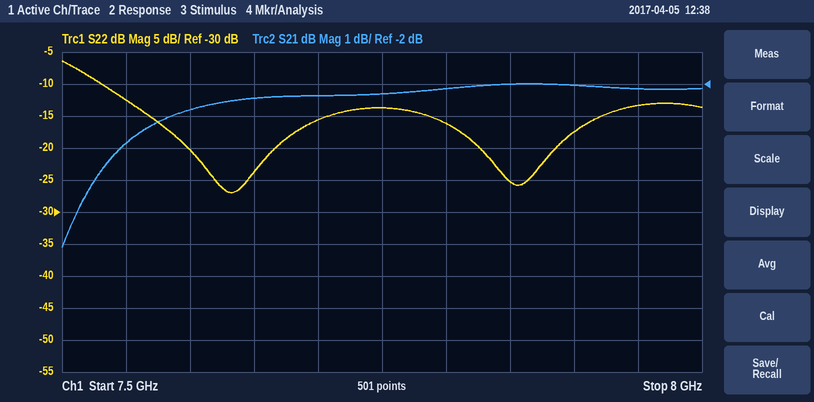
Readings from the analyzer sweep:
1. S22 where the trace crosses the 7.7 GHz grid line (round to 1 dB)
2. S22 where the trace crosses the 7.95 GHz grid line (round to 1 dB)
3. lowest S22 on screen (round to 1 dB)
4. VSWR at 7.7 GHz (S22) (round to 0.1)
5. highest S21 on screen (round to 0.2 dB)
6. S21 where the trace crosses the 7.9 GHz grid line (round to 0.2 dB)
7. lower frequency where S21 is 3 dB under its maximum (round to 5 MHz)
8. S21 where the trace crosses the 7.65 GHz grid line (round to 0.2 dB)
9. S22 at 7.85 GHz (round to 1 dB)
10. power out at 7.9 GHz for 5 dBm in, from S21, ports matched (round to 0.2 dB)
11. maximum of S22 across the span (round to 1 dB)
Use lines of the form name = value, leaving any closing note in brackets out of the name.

S22 where the trace crosses the 7.7 GHz grid line = -16 dB
S22 where the trace crosses the 7.95 GHz grid line = -13 dB
lowest S22 on screen = -27 dB
VSWR at 7.7 GHz (S22) = 1.4
highest S21 on screen = -2.0 dB
S21 where the trace crosses the 7.9 GHz grid line = -2.0 dB
lower frequency where S21 is 3 dB under its maximum = 7.525 GHz
S21 where the trace crosses the 7.65 GHz grid line = -2.4 dB
S22 at 7.85 GHz = -25 dB
power out at 7.9 GHz for 5 dBm in, from S21, ports matched = 3.0 dBm
maximum of S22 across the span = -6 dB
